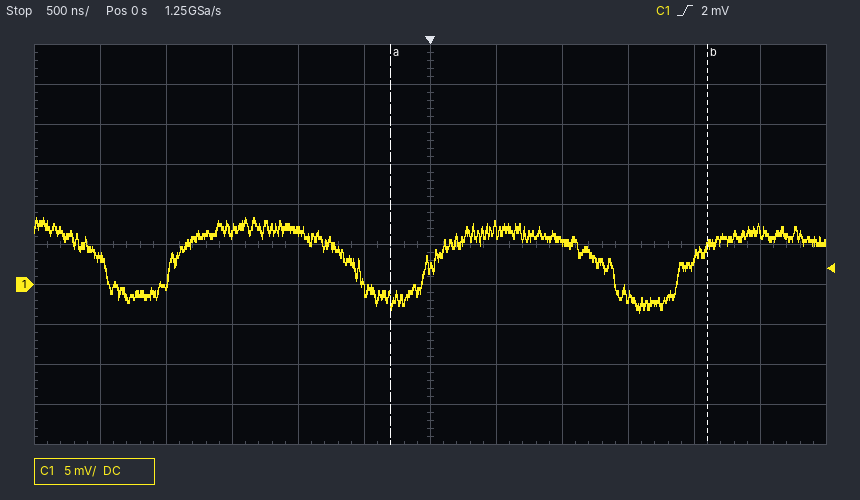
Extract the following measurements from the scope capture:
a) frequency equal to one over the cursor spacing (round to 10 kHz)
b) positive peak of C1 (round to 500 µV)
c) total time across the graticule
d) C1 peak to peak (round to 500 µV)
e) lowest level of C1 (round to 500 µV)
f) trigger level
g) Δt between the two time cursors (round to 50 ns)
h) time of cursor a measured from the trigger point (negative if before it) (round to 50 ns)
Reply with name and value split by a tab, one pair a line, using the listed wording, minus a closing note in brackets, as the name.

frequency equal to one over the cursor spacing	420 kHz
positive peak of C1	8.5 mV
total time across the graticule	6 µs
C1 peak to peak	12.0 mV
lowest level of C1	-3.5 mV
trigger level	2 mV
Δt between the two time cursors	2.40 µs
time of cursor a measured from the trigger point (negative if before it)	-300 ns
